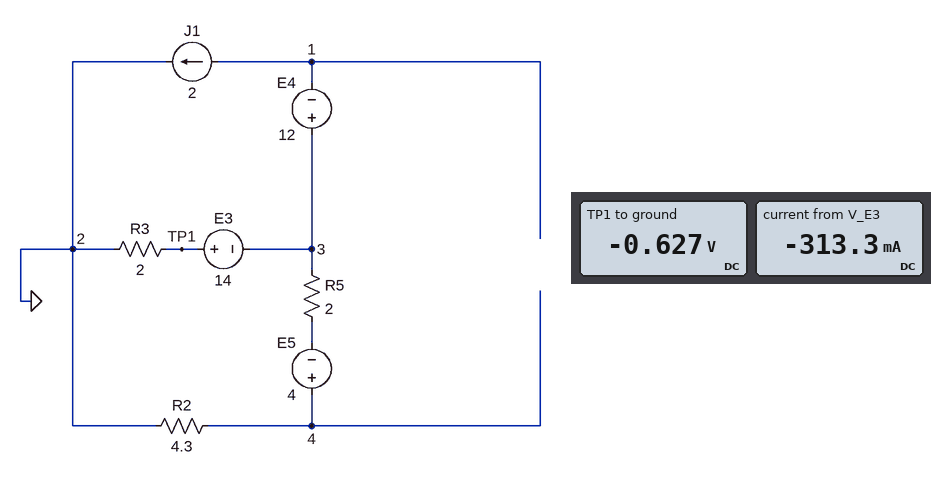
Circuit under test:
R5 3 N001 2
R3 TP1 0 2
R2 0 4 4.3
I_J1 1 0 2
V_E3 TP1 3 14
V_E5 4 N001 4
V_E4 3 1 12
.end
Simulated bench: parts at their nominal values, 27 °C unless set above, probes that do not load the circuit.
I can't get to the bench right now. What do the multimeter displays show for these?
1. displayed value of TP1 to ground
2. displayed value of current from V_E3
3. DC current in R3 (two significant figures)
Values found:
-0.627 V
-313.3 mA
310 mA
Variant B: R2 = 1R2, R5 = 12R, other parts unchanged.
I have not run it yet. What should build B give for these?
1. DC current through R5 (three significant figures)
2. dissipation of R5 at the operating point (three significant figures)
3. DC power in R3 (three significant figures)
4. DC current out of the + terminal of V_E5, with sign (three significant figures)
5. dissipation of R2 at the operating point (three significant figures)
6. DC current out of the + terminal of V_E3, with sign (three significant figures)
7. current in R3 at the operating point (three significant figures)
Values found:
921 mA
10.2 W
2.33 W
-921 mA
1.02 W
-1.08 A
1.08 A
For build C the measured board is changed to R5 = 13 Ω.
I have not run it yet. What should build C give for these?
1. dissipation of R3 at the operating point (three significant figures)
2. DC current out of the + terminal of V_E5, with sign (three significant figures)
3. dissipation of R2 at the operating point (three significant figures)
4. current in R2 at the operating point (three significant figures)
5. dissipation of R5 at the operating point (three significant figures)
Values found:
3.25 W
-725 mA
2.26 W
725 mA
6.84 W
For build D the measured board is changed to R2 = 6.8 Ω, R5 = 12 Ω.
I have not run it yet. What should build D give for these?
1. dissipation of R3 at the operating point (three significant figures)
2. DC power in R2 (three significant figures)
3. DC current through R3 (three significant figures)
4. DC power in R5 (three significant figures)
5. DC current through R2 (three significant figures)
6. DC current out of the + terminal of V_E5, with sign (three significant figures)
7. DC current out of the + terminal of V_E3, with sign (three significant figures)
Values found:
3.52 W
3.08 W
1.33 A
5.44 W
673 mA
-673 mA
-1.33 A
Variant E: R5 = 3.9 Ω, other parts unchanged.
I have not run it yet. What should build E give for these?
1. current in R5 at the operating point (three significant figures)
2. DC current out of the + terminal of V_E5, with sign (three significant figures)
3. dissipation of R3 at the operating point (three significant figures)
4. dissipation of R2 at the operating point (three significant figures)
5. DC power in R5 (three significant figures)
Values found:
1.37 A
-1.37 A
787 mW
8.10 W
7.35 W
